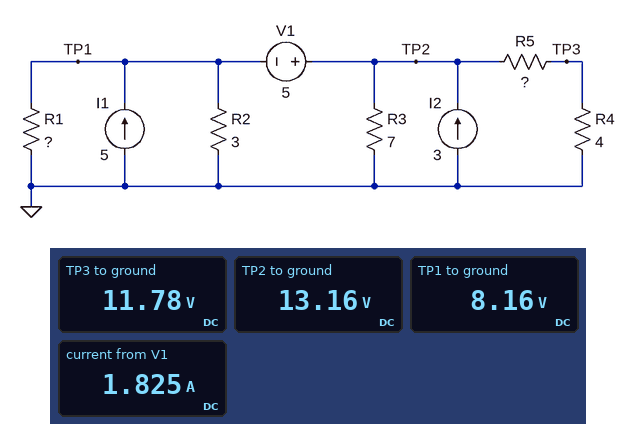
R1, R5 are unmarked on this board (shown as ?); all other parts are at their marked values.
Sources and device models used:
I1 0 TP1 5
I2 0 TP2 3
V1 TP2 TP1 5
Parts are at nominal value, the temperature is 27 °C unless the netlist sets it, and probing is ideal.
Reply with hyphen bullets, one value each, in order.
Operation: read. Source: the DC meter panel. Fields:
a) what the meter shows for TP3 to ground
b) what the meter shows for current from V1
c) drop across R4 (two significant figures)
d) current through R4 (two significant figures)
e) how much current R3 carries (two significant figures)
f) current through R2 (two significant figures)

- 11.78 V
- 1.825 A
- 12 V
- 2.9 A
- 1.9 A
- 2.7 A
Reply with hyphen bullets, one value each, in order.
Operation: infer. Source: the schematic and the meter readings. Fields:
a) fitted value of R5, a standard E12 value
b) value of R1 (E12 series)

- 0.47 Ω
- 18 Ω
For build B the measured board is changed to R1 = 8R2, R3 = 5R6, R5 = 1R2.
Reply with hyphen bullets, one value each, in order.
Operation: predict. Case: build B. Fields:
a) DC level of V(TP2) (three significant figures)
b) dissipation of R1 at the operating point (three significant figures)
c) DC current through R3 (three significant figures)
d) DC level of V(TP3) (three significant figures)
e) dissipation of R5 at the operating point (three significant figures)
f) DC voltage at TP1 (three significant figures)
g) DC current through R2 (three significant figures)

- 12.4 V
- 6.75 W
- 2.22 A
- 9.57 V
- 6.87 W
- 7.44 V
- 2.48 A
